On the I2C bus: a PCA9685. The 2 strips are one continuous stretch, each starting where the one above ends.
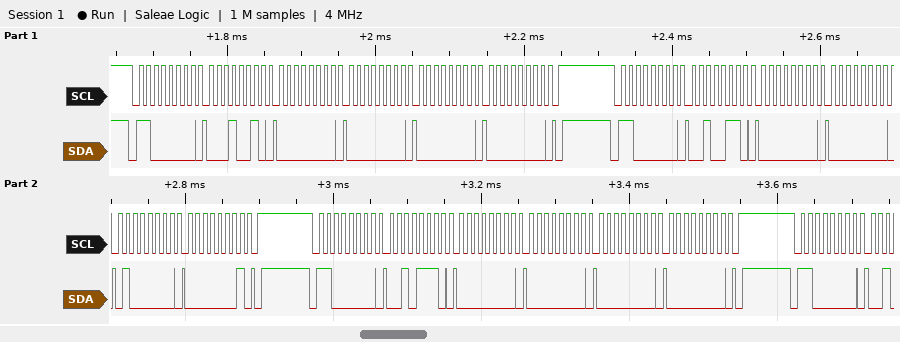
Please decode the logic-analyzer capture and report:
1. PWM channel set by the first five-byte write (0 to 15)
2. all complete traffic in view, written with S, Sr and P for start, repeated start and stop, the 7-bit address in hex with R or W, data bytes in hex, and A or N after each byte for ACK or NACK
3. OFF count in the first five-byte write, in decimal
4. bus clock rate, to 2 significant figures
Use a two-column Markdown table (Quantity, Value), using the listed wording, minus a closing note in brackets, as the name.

| Quantity | Value |
|---|---|
| PWM channel set by the first five-byte write | 3 |
| all complete traffic in view, written with S, Sr and P for start, repeated start and stop, the 7-bit address in hex with R or W, data bytes in hex, and A or N after each byte for ACK or NACK | S 60W A 12 A 00 A 00 A 00 A 00 A P S 60W A 26 A 00 A 00 A 40 A 01 A P S 60W A 2E A 00 A 00 A 00 A 00 A P S 60W A |
| OFF count in the first five-byte write, in decimal | 0 |
| bus clock rate, to 2 significant figures | 100 kHz |
